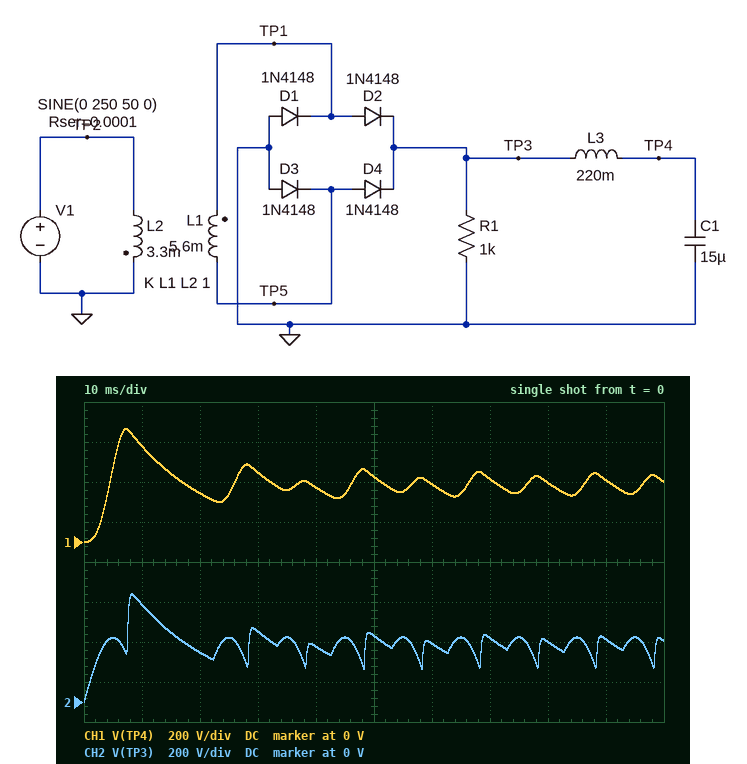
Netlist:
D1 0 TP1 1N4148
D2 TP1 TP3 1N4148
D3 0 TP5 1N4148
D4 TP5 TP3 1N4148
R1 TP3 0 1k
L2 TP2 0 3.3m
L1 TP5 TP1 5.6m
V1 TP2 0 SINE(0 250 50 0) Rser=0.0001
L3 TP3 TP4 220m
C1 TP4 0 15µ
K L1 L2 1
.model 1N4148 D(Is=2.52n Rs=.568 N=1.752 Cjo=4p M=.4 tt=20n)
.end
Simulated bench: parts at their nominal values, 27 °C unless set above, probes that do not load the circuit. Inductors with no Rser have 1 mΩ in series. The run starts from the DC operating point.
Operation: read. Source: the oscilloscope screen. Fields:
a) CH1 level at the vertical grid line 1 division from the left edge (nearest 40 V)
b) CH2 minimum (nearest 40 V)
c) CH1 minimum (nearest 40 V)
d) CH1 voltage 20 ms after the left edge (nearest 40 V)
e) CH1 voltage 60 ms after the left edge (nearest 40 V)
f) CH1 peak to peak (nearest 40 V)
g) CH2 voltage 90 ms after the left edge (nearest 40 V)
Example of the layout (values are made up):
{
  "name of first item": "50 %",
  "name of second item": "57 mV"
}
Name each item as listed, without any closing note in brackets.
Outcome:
{
  "CH1 level at the vertical grid line 1 division from the left edge": "480 V",
  "CH2 minimum": "0 V",
  "CH1 minimum": "0 V",
  "CH1 voltage 20 ms after the left edge": "240 V",
  "CH1 voltage 60 ms after the left edge": "280 V",
  "CH1 peak to peak": "560 V",
  "CH2 voltage 90 ms after the left edge": "320 V"
}
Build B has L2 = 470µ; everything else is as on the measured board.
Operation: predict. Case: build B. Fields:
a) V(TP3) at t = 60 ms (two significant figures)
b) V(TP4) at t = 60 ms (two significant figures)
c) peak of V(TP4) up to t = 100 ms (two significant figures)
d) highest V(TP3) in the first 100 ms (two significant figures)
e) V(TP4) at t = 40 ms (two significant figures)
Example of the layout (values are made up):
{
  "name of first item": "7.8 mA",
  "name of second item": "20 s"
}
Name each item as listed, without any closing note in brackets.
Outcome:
{
  "V(TP3) at t = 60 ms": "800 V",
  "V(TP4) at t = 60 ms": "790 V",
  "peak of V(TP4) up to t = 100 ms": "1.5 kV",
  "highest V(TP3) in the first 100 ms": "1.4 kV",
  "V(TP4) at t = 40 ms": "740 V"
}
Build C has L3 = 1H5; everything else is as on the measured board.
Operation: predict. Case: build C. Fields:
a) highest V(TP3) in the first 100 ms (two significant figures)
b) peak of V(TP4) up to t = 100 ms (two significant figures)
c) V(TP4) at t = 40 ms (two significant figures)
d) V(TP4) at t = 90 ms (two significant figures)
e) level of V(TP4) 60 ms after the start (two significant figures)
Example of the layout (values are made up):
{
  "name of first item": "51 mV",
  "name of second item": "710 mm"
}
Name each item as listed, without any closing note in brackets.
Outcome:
{
  "highest V(TP3) in the first 100 ms": "340 V",
  "peak of V(TP4) up to t = 100 ms": "410 V",
  "V(TP4) at t = 40 ms": "230 V",
  "V(TP4) at t = 90 ms": "220 V",
  "level of V(TP4) 60 ms after the start": "210 V"
}
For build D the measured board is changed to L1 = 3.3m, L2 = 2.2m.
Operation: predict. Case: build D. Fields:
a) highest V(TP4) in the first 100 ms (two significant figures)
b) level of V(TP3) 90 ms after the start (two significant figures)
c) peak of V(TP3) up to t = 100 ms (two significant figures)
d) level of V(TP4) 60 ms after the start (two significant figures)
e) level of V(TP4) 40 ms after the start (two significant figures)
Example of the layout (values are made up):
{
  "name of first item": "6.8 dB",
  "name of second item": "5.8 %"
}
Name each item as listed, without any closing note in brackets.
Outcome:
{
  "highest V(TP4) in the first 100 ms": "530 V",
  "level of V(TP3) 90 ms after the start": "290 V",
  "peak of V(TP3) up to t = 100 ms": "510 V",
  "level of V(TP4) 60 ms after the start": "270 V",
  "level of V(TP4) 40 ms after the start": "260 V"
}
